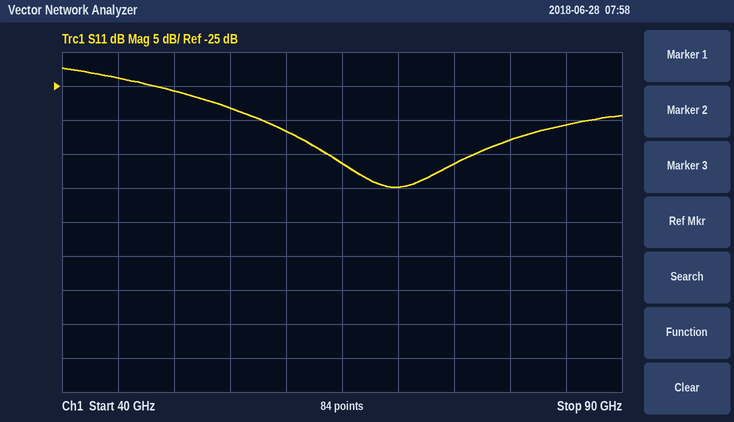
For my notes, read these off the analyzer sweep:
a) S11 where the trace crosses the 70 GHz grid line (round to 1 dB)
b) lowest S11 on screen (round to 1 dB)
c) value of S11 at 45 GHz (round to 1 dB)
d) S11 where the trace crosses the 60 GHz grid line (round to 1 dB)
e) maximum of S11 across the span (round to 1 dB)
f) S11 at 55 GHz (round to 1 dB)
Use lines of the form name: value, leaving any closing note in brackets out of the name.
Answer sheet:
S11 where the trace crosses the 70 GHz grid line: -40 dB
lowest S11 on screen: -40 dB
value of S11 at 45 GHz: -24 dB
S11 where the trace crosses the 60 GHz grid line: -32 dB
maximum of S11 across the span: -22 dB
S11 at 55 GHz: -28 dB
